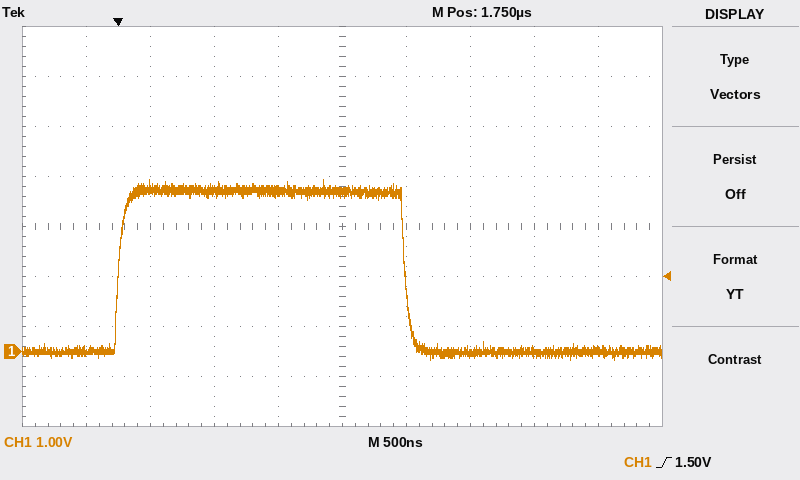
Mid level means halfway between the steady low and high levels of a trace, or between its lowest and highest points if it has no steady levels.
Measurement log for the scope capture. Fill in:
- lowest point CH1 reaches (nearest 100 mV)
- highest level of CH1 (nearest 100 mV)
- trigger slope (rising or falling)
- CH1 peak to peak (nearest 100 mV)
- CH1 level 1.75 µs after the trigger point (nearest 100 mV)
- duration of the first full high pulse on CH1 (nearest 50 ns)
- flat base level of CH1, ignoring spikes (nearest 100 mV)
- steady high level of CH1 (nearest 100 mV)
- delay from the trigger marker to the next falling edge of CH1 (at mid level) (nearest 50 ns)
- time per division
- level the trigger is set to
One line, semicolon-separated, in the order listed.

-200 mV; 3.4 V; rising; 3.6 V; 3.2 V; 2.25 µs; 0.0 V; 3.2 V; 2.25 µs; 500 ns; 1.50 V
